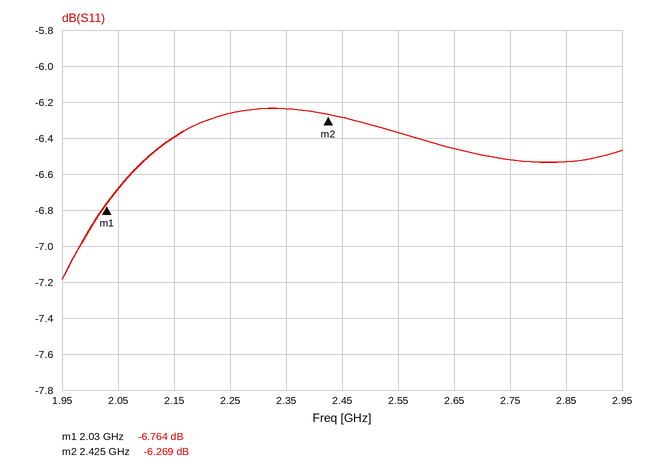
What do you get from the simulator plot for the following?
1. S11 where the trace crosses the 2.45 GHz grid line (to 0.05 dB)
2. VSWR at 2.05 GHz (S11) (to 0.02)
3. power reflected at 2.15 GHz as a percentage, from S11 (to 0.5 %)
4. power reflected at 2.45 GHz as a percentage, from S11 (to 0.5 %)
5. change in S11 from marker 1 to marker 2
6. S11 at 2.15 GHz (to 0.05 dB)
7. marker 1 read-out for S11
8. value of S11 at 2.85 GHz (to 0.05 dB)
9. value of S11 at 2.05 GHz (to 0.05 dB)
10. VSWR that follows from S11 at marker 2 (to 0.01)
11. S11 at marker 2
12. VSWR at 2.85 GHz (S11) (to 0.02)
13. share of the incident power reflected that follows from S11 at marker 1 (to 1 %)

-6.30 dB
2.72
23.0 %
23.5 %
0.495 dB
-6.40 dB
-6.764 dB
-6.55 dB
-6.70 dB
2.89
-6.269 dB
2.78
21 %
